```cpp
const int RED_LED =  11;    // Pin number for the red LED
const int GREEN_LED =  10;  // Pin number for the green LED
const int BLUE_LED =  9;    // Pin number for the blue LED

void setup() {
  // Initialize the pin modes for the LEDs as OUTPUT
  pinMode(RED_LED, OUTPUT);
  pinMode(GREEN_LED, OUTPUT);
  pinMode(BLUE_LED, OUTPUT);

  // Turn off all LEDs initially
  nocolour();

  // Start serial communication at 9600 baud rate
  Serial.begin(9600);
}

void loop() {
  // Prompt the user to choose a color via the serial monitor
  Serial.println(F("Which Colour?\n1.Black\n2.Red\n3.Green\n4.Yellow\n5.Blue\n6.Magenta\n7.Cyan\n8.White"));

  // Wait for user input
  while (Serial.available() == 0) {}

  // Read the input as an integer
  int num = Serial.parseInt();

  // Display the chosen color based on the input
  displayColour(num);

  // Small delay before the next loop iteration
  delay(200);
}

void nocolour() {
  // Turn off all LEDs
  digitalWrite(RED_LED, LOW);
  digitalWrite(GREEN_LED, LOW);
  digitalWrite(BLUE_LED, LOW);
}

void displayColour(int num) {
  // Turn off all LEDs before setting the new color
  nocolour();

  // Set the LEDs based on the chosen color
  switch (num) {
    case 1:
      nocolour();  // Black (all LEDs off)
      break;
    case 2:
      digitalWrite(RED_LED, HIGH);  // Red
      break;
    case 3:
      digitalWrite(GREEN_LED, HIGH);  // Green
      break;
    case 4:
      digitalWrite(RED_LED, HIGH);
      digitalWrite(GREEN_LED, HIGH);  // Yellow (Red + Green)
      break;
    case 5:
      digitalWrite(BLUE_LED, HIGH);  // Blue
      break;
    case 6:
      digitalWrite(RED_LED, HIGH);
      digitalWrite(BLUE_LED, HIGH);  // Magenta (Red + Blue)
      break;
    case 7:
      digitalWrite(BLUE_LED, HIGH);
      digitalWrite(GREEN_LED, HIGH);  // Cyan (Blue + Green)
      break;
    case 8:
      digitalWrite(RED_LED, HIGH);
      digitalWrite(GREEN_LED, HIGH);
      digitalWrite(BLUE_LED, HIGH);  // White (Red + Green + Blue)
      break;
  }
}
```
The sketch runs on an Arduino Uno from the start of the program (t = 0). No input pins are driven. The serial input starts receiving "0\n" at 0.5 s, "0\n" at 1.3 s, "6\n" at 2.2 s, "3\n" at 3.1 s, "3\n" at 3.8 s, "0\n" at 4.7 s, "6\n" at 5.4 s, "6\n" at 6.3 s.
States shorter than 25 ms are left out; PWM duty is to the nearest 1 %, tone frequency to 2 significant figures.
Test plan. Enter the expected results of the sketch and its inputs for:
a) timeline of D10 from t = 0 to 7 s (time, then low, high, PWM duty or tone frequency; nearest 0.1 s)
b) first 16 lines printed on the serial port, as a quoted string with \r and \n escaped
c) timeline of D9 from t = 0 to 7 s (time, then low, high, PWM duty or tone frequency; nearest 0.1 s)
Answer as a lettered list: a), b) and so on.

a) 0 s low; 3.1 s high; 4.7 s low
b) "Which Colour?\n1.Black\n2.Red\n3.Green\n4.Yellow\n5.Blue\n6.Magenta\n7.Cyan\n8.White\r\nWhich Colour?\n1.Black\n2.Red\n3.Green\n4.Yellow\n5.Blue\n6.Magenta\n"
c) 0 s low; 2.2 s high; 3.1 s low; 5.4 s high
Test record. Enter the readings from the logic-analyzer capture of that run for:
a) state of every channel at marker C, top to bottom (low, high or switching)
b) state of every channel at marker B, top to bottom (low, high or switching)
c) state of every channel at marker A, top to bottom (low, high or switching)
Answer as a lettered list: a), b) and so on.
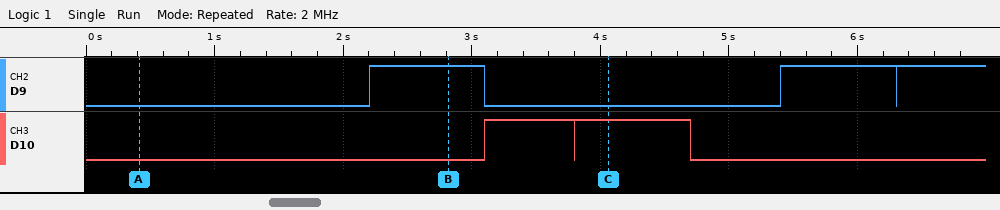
a) D9 low, D10 high
b) D9 high, D10 low
c) D9 low, D10 low
